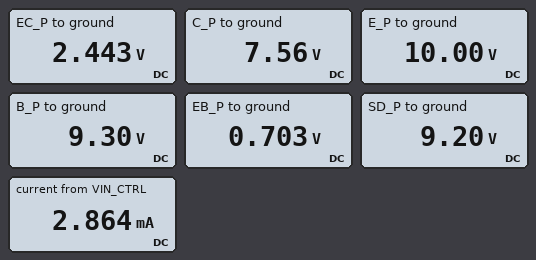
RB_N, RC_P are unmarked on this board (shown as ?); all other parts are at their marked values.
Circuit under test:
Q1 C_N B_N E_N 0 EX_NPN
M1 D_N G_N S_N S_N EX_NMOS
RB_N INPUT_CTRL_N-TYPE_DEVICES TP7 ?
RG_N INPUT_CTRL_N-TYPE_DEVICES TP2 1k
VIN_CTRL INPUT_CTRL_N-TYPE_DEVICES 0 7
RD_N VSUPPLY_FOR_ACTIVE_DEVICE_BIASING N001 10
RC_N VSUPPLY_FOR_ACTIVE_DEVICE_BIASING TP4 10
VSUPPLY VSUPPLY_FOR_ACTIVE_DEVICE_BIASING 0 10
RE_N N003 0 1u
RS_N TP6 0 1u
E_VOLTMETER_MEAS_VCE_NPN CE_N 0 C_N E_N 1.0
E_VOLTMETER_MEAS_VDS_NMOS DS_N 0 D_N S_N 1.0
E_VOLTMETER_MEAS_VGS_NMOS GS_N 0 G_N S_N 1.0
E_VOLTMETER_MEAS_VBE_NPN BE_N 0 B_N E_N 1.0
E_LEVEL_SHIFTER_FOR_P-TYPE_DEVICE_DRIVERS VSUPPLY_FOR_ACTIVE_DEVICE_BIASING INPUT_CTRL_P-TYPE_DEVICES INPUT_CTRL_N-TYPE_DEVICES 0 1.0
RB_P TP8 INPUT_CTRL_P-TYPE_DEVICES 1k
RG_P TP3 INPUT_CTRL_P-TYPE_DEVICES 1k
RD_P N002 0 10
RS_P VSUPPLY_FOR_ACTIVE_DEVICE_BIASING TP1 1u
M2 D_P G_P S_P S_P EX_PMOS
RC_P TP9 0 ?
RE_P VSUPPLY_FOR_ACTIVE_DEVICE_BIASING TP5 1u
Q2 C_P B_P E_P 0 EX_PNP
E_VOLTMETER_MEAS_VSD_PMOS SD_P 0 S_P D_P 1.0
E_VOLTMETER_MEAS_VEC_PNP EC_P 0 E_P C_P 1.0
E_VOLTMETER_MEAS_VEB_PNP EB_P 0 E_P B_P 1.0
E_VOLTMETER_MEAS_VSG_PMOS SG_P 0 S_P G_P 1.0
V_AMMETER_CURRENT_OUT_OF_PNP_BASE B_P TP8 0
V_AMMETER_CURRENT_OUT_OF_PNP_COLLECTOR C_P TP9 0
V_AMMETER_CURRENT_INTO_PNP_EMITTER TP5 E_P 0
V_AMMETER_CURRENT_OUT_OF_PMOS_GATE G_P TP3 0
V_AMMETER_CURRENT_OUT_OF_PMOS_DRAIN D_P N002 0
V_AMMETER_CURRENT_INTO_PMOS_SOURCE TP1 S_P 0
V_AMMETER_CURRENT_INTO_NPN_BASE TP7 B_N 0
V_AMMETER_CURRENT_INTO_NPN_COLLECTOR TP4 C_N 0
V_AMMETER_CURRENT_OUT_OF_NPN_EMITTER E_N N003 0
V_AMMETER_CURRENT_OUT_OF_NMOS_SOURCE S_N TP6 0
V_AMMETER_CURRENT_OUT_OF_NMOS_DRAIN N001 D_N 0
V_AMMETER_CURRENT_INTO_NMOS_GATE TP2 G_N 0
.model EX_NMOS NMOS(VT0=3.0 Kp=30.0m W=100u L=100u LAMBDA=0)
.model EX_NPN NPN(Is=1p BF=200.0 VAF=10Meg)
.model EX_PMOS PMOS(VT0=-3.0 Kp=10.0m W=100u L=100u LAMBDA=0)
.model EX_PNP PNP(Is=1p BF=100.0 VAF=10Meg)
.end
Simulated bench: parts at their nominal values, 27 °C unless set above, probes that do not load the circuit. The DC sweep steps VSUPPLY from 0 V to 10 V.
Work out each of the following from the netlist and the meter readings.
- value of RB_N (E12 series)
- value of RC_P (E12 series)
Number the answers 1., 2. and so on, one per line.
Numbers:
1. 2.2 kΩ
2. 12 Ω
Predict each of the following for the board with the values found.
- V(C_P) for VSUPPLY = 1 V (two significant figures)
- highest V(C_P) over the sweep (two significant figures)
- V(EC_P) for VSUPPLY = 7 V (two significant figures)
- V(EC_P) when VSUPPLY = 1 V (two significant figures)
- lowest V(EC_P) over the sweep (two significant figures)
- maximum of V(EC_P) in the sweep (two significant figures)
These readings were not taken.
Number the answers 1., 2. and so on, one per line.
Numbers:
1. 930 mV
2. 7.6 V
3. 180 mV
4. 72 mV
5. 15 mV
6. 2.4 V
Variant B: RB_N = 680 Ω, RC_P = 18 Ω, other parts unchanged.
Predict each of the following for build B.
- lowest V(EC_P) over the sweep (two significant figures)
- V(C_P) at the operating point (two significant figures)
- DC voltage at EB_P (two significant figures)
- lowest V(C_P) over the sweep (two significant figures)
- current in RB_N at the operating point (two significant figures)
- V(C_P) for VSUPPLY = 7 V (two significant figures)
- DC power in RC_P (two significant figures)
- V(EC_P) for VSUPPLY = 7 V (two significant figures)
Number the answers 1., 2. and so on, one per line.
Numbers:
1. 16 mV
2. 9.8 V
3. 700 mV
4. -16 mV
5. 9.2 mA
6. 6.9 V
7. 5.4 W
8. 130 mV
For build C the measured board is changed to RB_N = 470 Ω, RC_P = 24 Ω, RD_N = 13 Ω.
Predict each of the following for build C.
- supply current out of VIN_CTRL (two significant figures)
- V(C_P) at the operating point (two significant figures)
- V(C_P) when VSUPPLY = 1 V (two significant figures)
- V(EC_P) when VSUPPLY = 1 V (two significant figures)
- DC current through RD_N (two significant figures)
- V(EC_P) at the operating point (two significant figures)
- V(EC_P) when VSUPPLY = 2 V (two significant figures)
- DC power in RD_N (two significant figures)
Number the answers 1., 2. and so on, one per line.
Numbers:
1. 13 mA
2. 9.9 V
3. 940 mV
4. 56 mV
5. 240 mA
6. 140 mV
7. 73 mV
8. 750 mW
